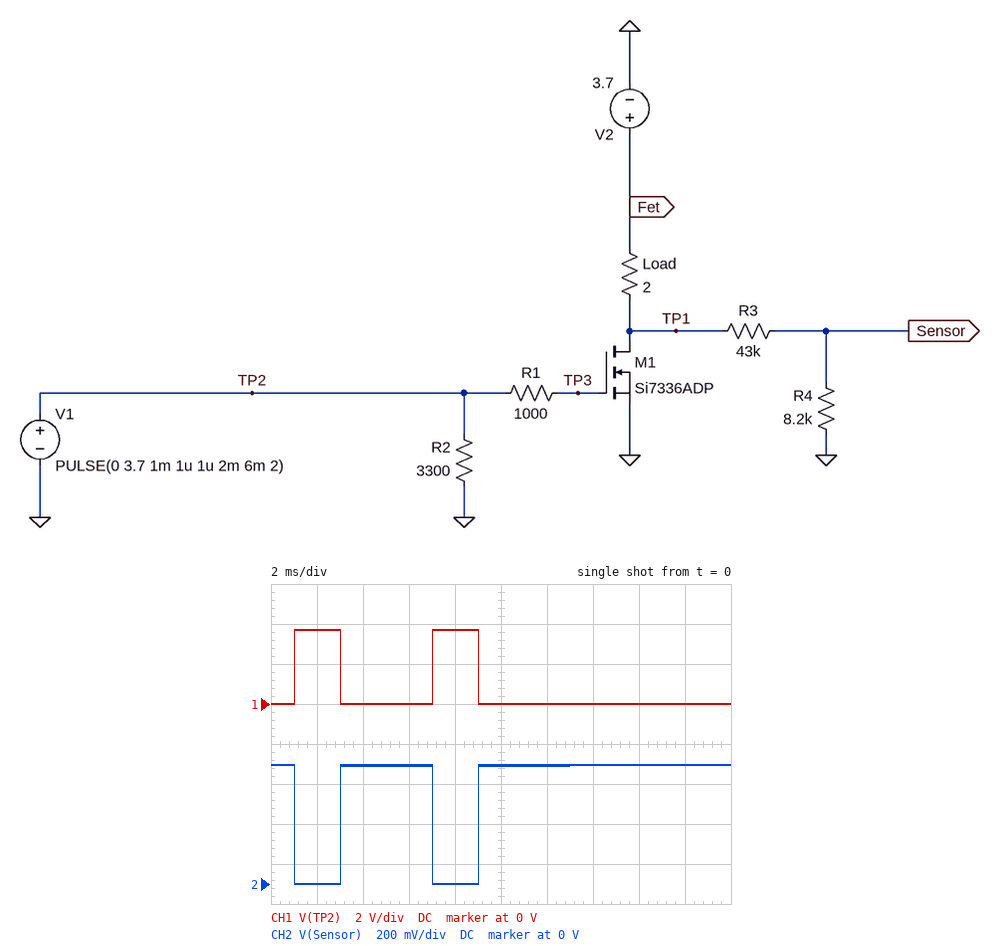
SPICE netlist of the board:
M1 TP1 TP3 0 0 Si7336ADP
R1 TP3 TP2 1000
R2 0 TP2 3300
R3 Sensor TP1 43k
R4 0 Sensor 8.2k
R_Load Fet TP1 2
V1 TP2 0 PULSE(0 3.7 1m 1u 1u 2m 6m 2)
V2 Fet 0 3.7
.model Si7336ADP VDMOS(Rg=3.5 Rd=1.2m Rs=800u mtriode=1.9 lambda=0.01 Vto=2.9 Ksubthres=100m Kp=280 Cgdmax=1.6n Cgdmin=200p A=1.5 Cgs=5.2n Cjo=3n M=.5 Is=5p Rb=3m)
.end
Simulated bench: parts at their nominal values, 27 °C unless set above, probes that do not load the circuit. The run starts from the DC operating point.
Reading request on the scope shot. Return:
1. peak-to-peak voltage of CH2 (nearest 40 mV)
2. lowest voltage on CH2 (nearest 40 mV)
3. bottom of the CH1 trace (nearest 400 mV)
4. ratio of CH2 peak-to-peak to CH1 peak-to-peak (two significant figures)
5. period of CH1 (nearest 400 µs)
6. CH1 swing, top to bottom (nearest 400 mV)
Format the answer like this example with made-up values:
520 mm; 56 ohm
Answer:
600 mV; 0 V; 0 V; 0.16; 6.0 ms; 3.6 V
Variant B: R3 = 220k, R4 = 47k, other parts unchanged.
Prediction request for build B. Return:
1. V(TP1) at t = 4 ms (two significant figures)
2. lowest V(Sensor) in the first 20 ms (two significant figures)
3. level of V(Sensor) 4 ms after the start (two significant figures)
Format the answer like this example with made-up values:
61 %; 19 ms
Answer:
3.7 V; 1.4 mV; 650 mV
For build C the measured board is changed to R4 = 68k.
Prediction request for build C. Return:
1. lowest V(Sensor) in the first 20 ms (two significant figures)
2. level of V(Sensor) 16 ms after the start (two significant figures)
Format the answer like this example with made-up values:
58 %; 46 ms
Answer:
4.9 mV; 2.3 V
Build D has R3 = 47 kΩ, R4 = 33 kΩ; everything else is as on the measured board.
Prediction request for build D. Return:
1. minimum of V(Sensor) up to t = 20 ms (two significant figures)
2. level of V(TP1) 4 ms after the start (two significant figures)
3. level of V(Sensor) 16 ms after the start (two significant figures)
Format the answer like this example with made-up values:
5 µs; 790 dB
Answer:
3.3 mV; 3.7 V; 1.5 V
